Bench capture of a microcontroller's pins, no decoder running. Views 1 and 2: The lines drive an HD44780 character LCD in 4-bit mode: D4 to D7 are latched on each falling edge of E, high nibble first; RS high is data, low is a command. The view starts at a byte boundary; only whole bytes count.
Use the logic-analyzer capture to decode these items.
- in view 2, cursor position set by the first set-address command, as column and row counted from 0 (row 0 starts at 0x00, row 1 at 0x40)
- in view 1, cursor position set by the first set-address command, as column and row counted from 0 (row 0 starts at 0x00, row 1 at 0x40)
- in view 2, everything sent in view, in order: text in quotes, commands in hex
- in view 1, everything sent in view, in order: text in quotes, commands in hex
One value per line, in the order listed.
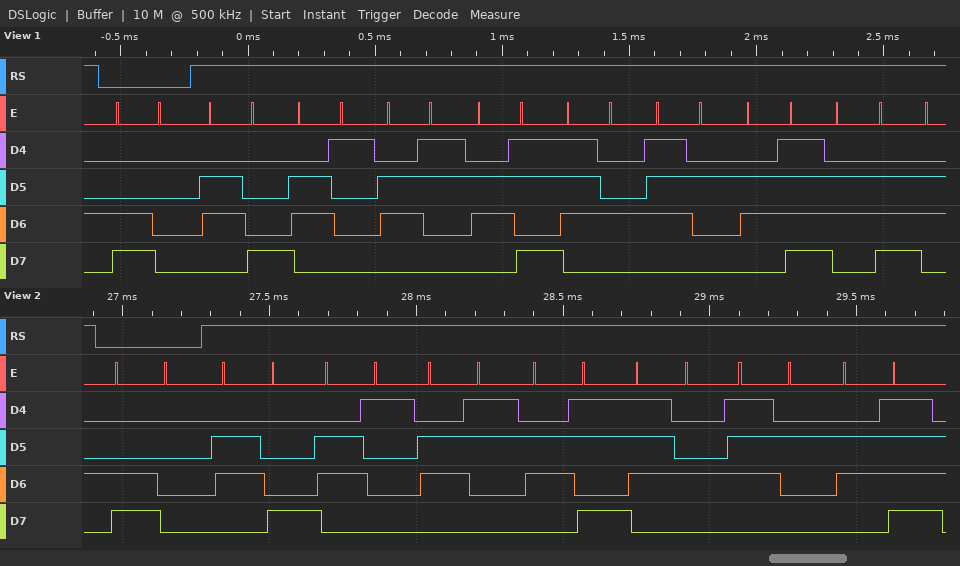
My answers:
column 0, row 1
column 0, row 1
0xC0 "hacktro"
0xC0 "hacktron"
